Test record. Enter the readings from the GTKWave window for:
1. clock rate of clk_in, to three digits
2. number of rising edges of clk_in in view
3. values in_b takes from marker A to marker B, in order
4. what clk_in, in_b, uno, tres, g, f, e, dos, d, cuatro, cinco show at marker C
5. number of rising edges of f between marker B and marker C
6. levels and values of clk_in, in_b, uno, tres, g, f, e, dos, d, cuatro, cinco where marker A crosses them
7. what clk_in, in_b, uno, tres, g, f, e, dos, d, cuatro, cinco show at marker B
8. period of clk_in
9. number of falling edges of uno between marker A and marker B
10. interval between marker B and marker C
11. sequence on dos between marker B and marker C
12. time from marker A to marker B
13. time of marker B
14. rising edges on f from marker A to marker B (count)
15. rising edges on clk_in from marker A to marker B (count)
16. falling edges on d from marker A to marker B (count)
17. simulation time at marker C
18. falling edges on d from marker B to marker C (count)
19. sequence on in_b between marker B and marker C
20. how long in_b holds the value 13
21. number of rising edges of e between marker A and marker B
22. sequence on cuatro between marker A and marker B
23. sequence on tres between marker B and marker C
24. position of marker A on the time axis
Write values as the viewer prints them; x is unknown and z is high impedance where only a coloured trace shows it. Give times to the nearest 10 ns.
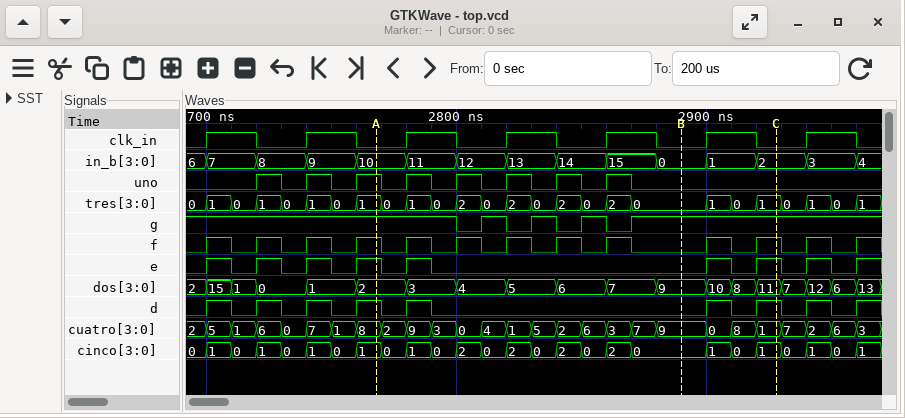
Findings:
25.0 MHz
7
10, 11, 12, 13, 14, 15, 0
clk_in=0, in_b=2, uno=0, tres=1, g=1, f=1, e=1, dos=11, d=1, cuatro=1, cinco=1
2
clk_in=0, in_b=10, uno=1, tres=1, g=1, f=1, e=1, dos=2, d=1, cuatro=8, cinco=1
clk_in=0, in_b=0, uno=0, tres=0, g=1, f=0, e=0, dos=9, d=0, cuatro=9, cinco=0
40 ns
6
40 ns
9, 10, 8, 11
120 ns
2890 ns
5
3
2
2930 ns
1
0, 1, 2
20 ns
1
8, 2, 9, 3, 0, 4, 1, 5, 2, 6, 3, 7, 9
0, 1, 0, 1
2770 ns
